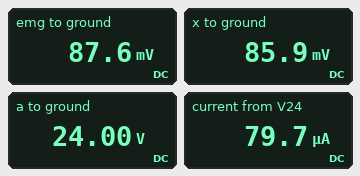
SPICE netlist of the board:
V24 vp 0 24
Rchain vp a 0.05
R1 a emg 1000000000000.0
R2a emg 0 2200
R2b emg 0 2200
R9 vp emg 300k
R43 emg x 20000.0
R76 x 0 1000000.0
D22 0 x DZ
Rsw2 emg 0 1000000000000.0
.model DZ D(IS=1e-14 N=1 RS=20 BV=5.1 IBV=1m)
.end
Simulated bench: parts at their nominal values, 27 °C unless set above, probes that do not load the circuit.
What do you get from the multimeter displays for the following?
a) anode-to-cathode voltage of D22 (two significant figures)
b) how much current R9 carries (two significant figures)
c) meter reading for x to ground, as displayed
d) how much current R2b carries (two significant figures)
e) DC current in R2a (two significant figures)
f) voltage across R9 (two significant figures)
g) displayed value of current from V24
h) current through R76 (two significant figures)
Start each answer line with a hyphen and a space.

- -86 mV
- 80 µA
- 85.9 mV
- 40 µA
- 40 µA
- 24 V
- 79.7 µA
- 86 nA
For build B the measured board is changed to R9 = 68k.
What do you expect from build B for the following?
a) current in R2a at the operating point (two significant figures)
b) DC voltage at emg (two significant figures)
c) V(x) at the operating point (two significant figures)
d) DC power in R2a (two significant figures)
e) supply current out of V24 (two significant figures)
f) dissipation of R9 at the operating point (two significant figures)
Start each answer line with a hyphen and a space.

- 170 µA
- 380 mV
- 370 mV
- 66 µW
- 350 µA
- 8.2 mW
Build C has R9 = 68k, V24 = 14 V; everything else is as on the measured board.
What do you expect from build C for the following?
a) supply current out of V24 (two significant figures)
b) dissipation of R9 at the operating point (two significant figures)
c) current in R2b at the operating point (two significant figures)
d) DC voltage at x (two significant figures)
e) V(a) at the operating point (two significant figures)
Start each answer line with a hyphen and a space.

- 200 µA
- 2.8 mW
- 100 µA
- 220 mV
- 14 V
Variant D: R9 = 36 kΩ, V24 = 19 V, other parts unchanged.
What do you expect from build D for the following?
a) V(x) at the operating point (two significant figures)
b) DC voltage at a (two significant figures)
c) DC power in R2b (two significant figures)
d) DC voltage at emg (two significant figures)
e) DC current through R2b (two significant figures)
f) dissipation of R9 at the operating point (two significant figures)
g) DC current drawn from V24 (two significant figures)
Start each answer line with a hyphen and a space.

- 550 mV
- 19 V
- 140 µW
- 560 mV
- 260 µA
- 9.4 mW
- 510 µA
